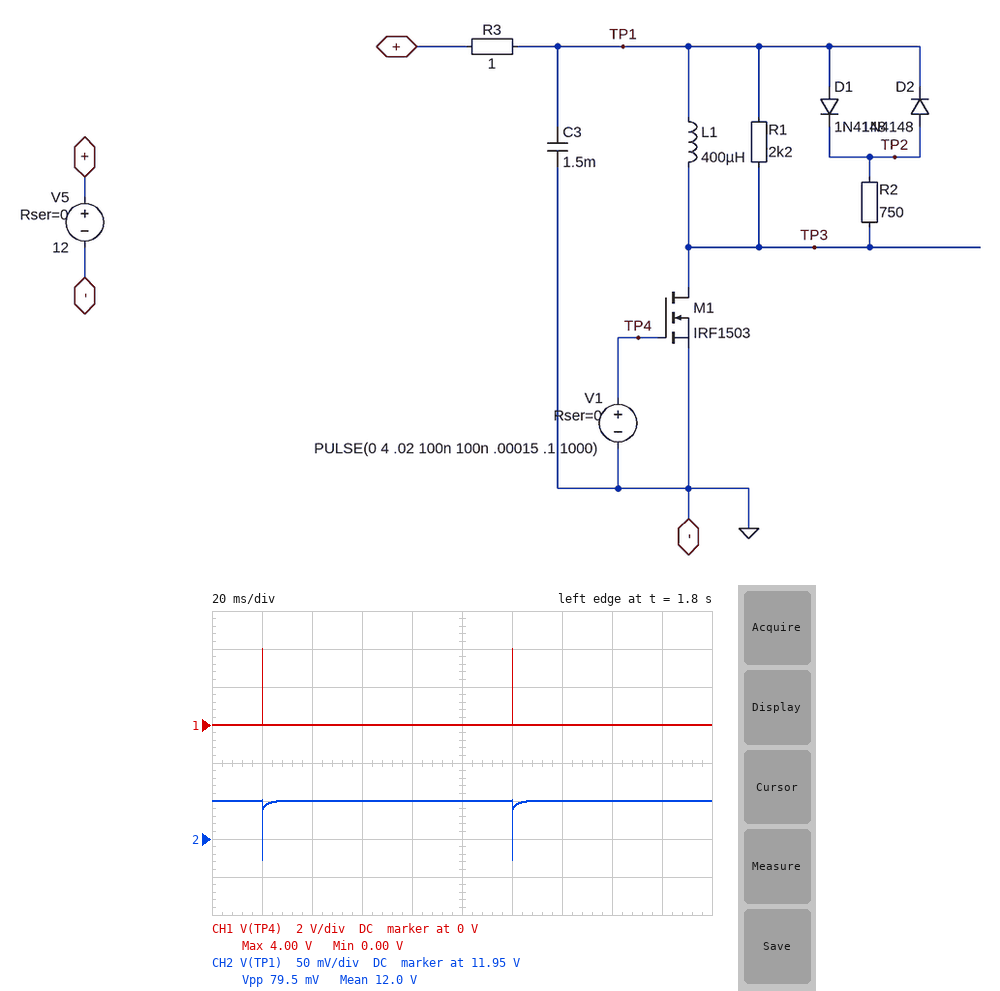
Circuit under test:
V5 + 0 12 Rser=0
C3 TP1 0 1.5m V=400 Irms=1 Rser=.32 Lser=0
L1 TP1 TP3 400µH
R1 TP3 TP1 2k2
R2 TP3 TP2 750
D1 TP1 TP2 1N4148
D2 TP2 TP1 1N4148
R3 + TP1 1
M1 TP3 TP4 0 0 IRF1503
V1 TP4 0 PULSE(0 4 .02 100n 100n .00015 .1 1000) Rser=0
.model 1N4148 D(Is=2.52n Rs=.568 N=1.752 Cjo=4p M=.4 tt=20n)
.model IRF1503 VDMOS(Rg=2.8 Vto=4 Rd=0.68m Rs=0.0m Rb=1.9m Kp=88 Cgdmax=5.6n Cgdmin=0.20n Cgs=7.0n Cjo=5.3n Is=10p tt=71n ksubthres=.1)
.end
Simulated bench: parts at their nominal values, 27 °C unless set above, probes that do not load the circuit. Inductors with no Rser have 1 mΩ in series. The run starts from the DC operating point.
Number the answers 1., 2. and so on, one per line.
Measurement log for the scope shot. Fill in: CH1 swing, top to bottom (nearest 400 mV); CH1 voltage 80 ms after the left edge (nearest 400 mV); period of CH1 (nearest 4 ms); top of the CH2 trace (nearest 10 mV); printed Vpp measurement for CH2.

1. 4.0 V
2. 0 V
3. 100 ms
4. 12.00 V
5. 79.5 mV
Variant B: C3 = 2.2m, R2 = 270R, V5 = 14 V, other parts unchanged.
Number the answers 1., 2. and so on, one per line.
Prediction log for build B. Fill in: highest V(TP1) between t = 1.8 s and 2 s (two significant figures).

1. 14 V
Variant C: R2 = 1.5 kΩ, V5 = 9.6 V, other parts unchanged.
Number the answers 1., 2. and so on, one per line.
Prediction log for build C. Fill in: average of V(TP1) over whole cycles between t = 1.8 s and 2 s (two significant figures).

1. 9.6 V
